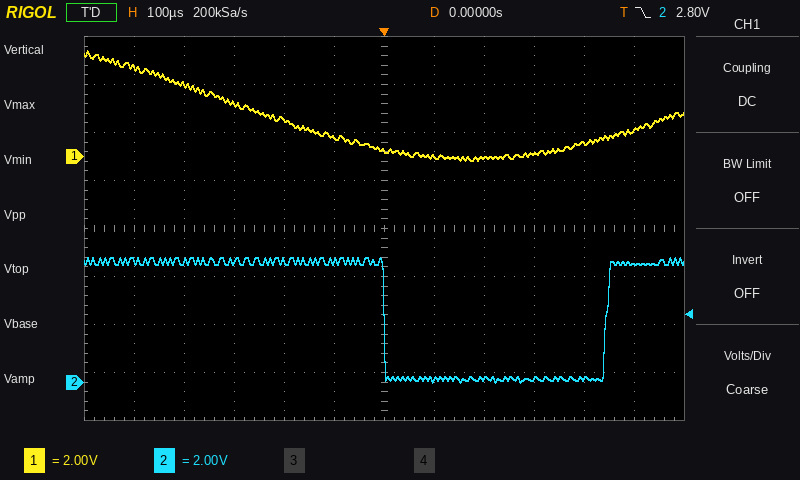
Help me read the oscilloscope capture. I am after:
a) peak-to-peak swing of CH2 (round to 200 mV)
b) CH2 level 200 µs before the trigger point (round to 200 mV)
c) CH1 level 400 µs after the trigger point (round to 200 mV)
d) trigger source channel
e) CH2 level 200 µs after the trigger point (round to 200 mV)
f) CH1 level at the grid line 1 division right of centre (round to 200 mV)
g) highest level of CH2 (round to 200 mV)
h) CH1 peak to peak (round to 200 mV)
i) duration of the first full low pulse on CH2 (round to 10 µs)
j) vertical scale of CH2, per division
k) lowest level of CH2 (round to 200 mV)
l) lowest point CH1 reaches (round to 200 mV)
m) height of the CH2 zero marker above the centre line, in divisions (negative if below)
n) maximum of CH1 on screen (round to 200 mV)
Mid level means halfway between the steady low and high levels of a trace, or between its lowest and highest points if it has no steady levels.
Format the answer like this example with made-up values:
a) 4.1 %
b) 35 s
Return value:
a) 5.2 V
b) 5.0 V
c) 600 mV
d) CH2
e) 200 mV
f) 0.0 V
g) 5.2 V
h) 4.6 V
i) 440 µs
j) 2 V
k) 0.0 V
l) -200 mV
m) -3.2 div
n) 4.4 V
